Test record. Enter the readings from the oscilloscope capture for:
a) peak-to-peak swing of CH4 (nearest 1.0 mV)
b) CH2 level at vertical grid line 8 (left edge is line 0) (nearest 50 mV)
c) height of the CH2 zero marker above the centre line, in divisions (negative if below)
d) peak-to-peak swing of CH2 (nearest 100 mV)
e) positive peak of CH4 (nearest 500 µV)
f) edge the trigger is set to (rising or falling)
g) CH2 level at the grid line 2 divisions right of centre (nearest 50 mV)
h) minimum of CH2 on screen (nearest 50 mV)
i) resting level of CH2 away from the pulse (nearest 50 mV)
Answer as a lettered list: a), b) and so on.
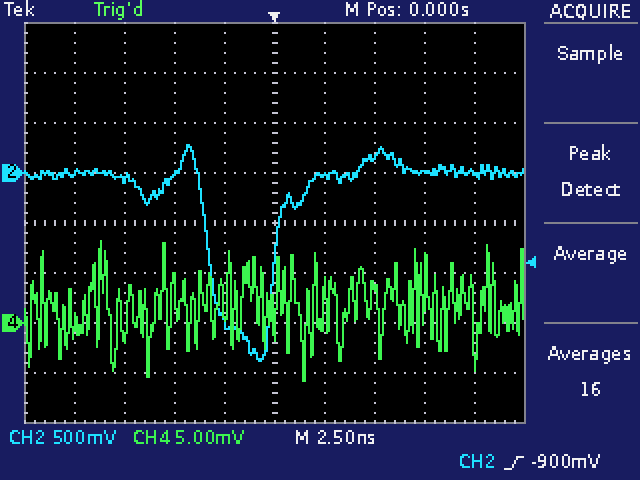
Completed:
a) 14.0 mV
b) 0 mV
c) +1.0 div
d) 2.20 V
e) 8.0 mV
f) rising
g) 150 mV
h) -1.90 V
i) 0 mV
